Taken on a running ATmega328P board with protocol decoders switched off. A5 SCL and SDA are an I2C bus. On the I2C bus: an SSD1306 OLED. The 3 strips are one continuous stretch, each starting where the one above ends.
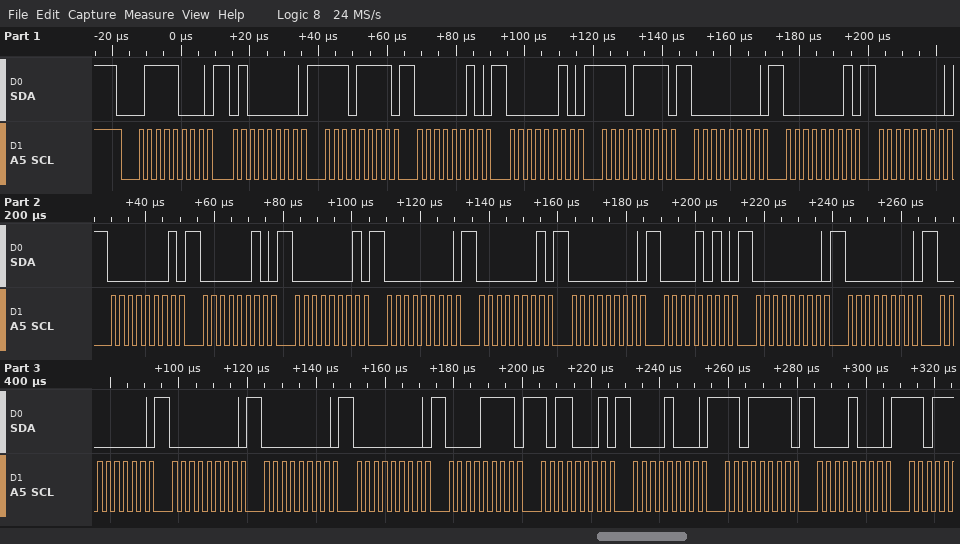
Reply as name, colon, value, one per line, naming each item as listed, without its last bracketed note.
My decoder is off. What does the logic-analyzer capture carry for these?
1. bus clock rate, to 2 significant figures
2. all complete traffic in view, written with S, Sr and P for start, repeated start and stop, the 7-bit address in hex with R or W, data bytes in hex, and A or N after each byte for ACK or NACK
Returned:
bus clock rate, to 2 significant figures: 400 kHz
all complete traffic in view, written with S, Sr and P for start, repeated start and stop, the 7-bit address in hex with R or W, data bytes in hex, and A or N after each byte for ACK or NACK: S 3CW A 40 A EF A 02 A 02 A EF A 00 A 01 A 00 A 01 A 02 A 01 A 00 A 01 A 00 A 0A A 00 A 00 A 00 A 00 A 00 A 00 A 0F A B1 A 08 A DF A 08 A
